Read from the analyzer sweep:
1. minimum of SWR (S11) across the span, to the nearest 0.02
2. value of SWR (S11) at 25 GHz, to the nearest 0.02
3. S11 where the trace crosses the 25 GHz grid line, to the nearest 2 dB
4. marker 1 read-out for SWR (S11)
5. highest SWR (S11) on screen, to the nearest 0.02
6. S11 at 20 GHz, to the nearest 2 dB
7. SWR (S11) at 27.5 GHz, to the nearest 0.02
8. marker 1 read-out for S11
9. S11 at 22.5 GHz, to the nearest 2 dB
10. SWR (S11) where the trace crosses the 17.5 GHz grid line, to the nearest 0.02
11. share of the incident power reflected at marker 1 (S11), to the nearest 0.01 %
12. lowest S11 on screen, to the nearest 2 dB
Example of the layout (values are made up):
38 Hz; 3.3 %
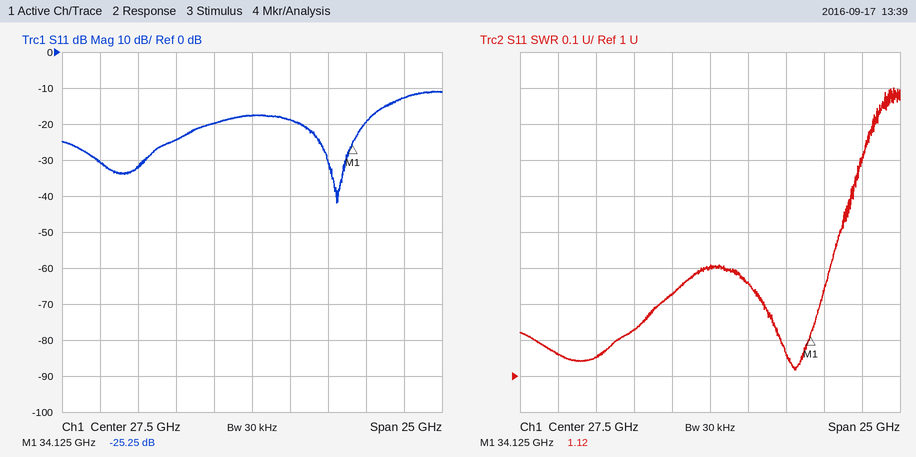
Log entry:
1.02; 1.22; -20 dB; 1.12; 1.80; -32 dB; 1.30; -25.25 dB; -24 dB; 1.06; 0.30 %; -42 dB
